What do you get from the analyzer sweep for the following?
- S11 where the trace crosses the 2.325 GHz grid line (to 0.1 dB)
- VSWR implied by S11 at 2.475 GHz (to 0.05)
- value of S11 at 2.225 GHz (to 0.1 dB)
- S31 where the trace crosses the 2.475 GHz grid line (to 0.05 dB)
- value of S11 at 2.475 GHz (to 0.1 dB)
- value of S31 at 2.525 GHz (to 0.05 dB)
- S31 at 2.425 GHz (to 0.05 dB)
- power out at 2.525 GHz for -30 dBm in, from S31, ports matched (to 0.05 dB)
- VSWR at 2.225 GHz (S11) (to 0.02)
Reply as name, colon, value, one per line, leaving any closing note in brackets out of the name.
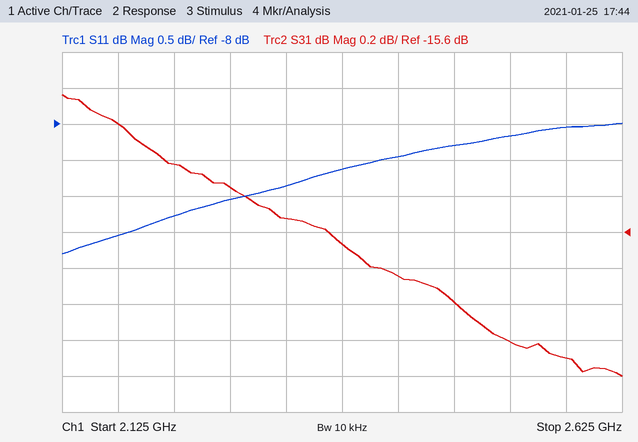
S11 where the trace crosses the 2.325 GHz grid line: -8.9 dB
VSWR implied by S11 at 2.475 GHz: 2.25
value of S11 at 2.225 GHz: -9.3 dB
S31 where the trace crosses the 2.475 GHz grid line: -16.00 dB
value of S11 at 2.475 GHz: -8.3 dB
value of S31 at 2.525 GHz: -16.20 dB
S31 at 2.425 GHz: -15.85 dB
power out at 2.525 GHz for -30 dBm in, from S31, ports matched: -46.20 dBm
VSWR at 2.225 GHz (S11): 2.04
